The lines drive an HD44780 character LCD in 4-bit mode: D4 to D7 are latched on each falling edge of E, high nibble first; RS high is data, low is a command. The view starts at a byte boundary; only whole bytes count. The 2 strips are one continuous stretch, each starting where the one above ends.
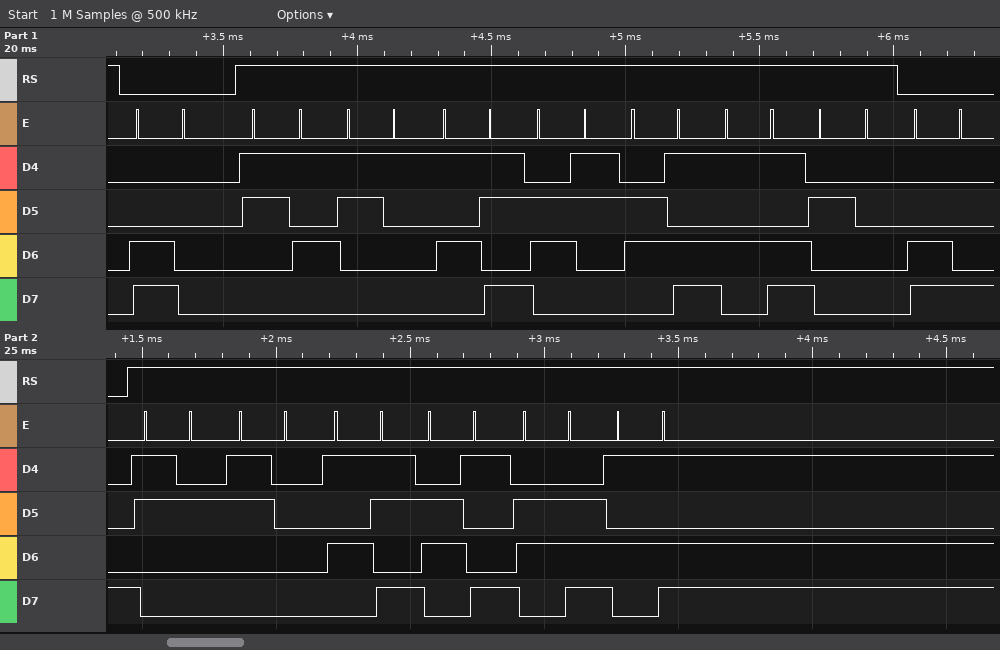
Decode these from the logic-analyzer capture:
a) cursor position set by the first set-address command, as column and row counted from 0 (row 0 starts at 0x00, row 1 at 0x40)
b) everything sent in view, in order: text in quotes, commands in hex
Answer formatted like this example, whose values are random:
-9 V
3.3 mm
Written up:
column 0, row 1
0xC0 "51[cm] " 0xC8 "20[in]"
